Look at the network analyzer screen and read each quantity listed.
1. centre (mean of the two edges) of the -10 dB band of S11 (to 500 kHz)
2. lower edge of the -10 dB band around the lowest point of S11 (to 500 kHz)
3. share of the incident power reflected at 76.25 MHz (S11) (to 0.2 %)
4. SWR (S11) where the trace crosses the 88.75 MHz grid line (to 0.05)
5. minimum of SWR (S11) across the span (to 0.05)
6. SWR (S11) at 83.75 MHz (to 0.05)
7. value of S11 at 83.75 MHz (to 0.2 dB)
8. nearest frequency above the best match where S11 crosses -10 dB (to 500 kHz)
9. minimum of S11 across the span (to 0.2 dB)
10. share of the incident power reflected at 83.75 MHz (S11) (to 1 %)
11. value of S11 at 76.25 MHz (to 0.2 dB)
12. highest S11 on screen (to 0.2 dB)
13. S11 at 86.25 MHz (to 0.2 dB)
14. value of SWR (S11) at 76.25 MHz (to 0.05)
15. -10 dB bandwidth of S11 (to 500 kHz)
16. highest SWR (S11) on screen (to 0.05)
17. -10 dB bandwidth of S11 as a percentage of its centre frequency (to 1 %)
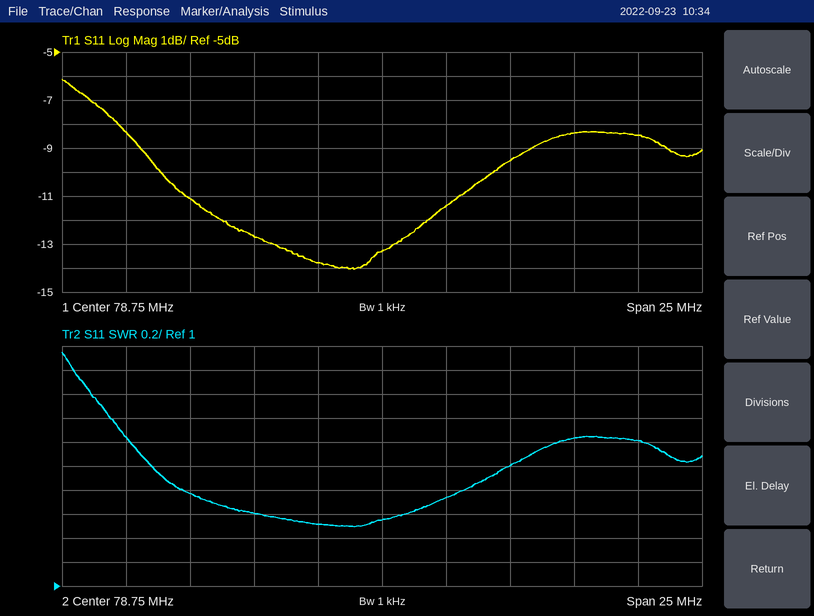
76.5 MHz
70.0 MHz
4.2 %
2.20
1.50
2.00
-9.6 dB
83.0 MHz
-14.0 dB
11 %
-13.8 dB
-6.2 dB
-8.4 dB
1.50
13.0 MHz
2.95
17 %
